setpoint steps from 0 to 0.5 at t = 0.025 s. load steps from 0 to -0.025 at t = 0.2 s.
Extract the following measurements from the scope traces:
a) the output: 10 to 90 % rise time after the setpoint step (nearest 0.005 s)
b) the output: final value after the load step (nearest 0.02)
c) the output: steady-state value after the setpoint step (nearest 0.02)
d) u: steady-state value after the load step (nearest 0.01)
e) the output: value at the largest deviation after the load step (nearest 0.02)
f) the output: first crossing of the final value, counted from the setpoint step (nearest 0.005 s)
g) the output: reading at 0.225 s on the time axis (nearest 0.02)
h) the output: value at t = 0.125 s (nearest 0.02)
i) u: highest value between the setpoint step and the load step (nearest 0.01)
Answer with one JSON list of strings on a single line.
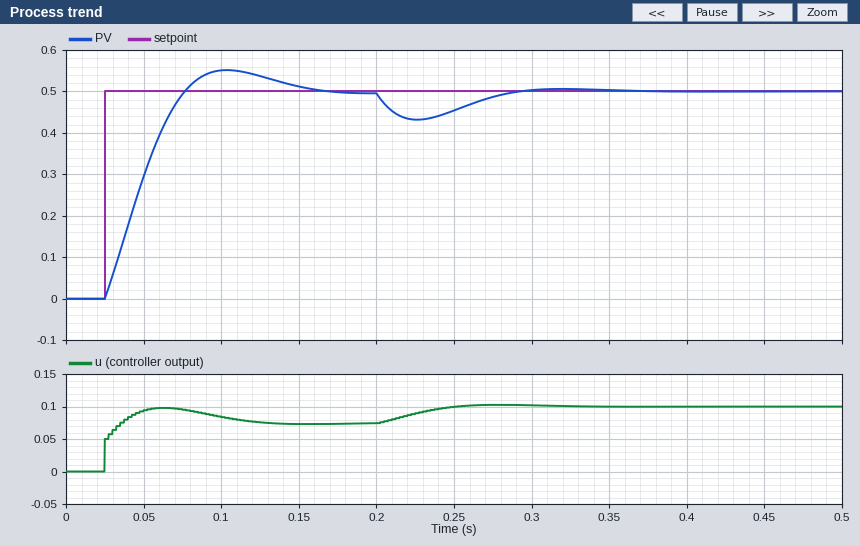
["0.040 s", "0.50", "0.50", "0.10", "0.44", "0.050 s", "0.44", "0.54", "0.10"]
